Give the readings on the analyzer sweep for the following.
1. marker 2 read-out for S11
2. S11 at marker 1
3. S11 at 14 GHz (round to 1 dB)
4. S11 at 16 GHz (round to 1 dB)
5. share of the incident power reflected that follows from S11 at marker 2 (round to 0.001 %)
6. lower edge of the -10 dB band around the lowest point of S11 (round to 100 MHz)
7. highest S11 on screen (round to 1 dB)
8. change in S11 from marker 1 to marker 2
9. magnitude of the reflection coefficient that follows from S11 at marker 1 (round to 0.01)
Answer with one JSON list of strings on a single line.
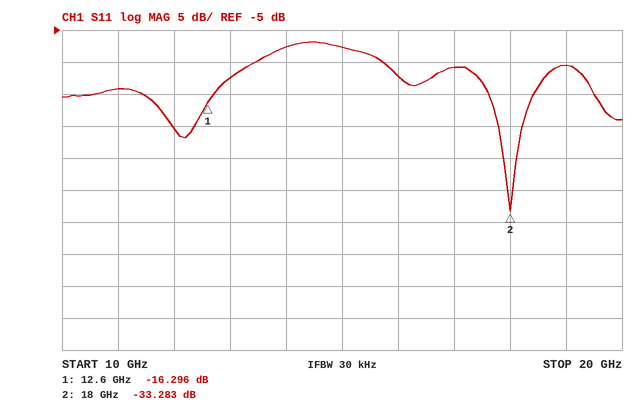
["-33.283 dB", "-16.296 dB", "-8 dB", "-12 dB", "0.047 %", "15.7 GHz", "-7 dB", "-16.987 dB", "0.15"]
